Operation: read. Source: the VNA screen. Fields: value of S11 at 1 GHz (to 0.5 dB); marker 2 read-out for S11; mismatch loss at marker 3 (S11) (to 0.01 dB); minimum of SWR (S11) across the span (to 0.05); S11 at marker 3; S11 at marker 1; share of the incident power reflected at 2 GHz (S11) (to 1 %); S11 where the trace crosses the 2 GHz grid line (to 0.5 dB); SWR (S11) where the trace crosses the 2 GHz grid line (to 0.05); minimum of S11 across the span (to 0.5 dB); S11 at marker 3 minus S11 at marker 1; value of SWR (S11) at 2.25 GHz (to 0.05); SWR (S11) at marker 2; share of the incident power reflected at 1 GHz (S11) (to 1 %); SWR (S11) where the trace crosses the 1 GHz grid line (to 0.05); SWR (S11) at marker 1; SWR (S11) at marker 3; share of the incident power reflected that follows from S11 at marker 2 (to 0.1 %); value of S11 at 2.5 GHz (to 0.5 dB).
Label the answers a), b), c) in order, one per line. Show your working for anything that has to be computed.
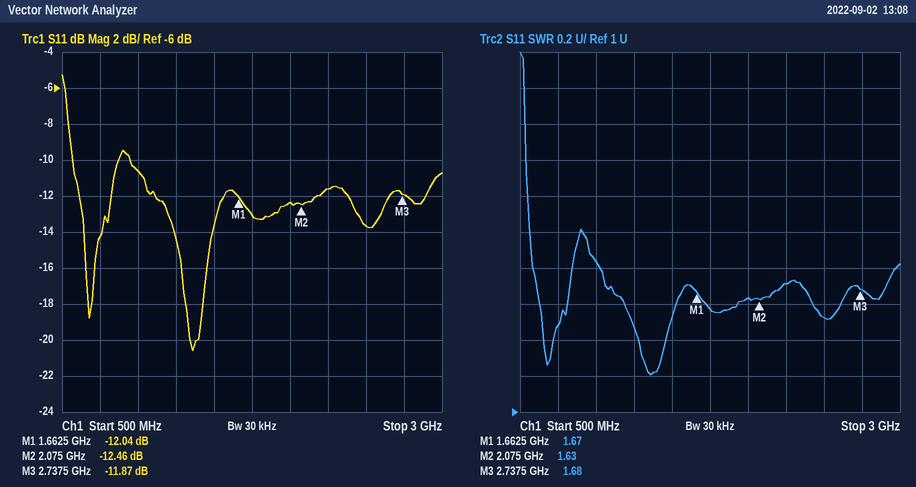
a) -10.5 dB
b) -12.46 dB
c) −10 log10(1 − 10^(-11.87/10)) ≈ 0.29 dB
d) 1.20
e) -11.87 dB
f) -12.04 dB
g) 10^(-12.5/10) ≈ 6 %
h) -12.5 dB
i) 1.65
j) -20.5 dB
k) -11.87 − (-12.04) = 0.17 dB
l) 1.70
m) 1.63
n) 10^(-10.5/10) ≈ 9 %
o) 1.85
p) 1.67
q) 1.68
r) 10^(-12.46/10) ≈ 5.7 %
s) -13.5 dB
